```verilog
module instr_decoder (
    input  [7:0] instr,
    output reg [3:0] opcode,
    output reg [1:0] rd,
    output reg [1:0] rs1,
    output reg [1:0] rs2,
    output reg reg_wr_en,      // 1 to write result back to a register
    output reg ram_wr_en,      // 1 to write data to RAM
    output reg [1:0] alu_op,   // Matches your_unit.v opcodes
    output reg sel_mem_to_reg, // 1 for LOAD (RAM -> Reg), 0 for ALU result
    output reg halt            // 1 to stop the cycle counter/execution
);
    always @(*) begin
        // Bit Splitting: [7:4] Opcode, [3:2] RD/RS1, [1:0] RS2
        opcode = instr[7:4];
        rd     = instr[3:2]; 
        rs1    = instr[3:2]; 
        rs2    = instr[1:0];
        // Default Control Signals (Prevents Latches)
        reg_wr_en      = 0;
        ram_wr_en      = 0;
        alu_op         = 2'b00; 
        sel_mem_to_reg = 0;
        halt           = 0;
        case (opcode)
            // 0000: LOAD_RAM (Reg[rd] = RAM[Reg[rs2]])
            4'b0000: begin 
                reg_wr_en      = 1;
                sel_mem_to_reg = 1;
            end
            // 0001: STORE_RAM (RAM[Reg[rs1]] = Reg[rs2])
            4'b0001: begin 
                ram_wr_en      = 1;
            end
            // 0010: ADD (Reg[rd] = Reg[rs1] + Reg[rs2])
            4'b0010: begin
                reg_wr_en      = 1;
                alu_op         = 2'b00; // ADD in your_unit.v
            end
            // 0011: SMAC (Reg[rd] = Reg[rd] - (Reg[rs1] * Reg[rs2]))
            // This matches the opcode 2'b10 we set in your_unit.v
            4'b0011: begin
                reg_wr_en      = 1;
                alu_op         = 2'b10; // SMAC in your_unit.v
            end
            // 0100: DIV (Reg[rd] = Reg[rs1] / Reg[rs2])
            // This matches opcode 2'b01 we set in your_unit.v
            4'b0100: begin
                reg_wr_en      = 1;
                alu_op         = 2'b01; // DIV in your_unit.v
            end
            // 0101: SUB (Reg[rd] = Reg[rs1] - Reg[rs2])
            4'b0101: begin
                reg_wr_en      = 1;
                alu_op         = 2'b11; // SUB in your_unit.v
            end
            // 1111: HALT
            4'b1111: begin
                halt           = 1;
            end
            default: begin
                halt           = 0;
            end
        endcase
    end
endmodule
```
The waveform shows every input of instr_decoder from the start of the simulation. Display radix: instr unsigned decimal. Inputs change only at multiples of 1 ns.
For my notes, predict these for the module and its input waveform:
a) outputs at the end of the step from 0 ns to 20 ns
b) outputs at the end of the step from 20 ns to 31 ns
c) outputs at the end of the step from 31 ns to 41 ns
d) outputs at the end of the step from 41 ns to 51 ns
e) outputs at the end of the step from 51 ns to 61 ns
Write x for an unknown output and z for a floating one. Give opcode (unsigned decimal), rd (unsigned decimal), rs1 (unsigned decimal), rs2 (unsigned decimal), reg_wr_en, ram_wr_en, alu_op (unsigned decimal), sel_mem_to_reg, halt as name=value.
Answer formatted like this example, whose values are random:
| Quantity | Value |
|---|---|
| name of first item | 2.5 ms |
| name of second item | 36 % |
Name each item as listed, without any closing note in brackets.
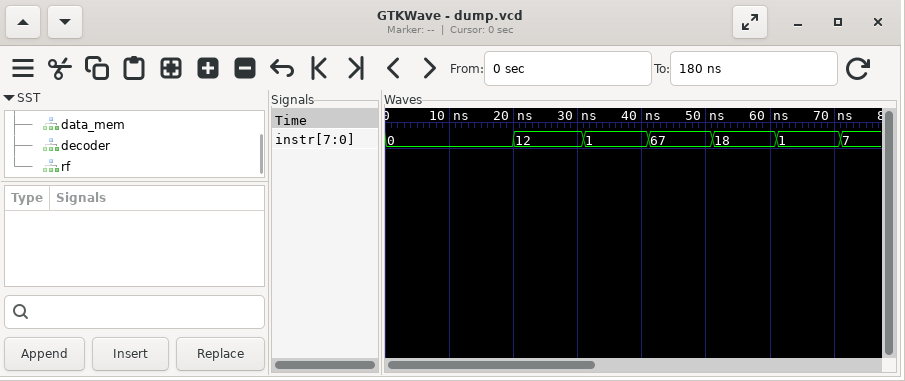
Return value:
| Quantity | Value |
|---|---|
| outputs at the end of the step from 0 ns to 20 ns | opcode=0, rd=0, rs1=0, rs2=0, reg_wr_en=1, ram_wr_en=0, alu_op=0, sel_mem_to_reg=1, halt=0 |
| outputs at the end of the step from 20 ns to 31 ns | opcode=0, rd=3, rs1=3, rs2=0, reg_wr_en=1, ram_wr_en=0, alu_op=0, sel_mem_to_reg=1, halt=0 |
| outputs at the end of the step from 31 ns to 41 ns | opcode=0, rd=0, rs1=0, rs2=1, reg_wr_en=1, ram_wr_en=0, alu_op=0, sel_mem_to_reg=1, halt=0 |
| outputs at the end of the step from 41 ns to 51 ns | opcode=4, rd=0, rs1=0, rs2=3, reg_wr_en=1, ram_wr_en=0, alu_op=1, sel_mem_to_reg=0, halt=0 |
| outputs at the end of the step from 51 ns to 61 ns | opcode=1, rd=0, rs1=0, rs2=2, reg_wr_en=0, ram_wr_en=1, alu_op=0, sel_mem_to_reg=0, halt=0 |
